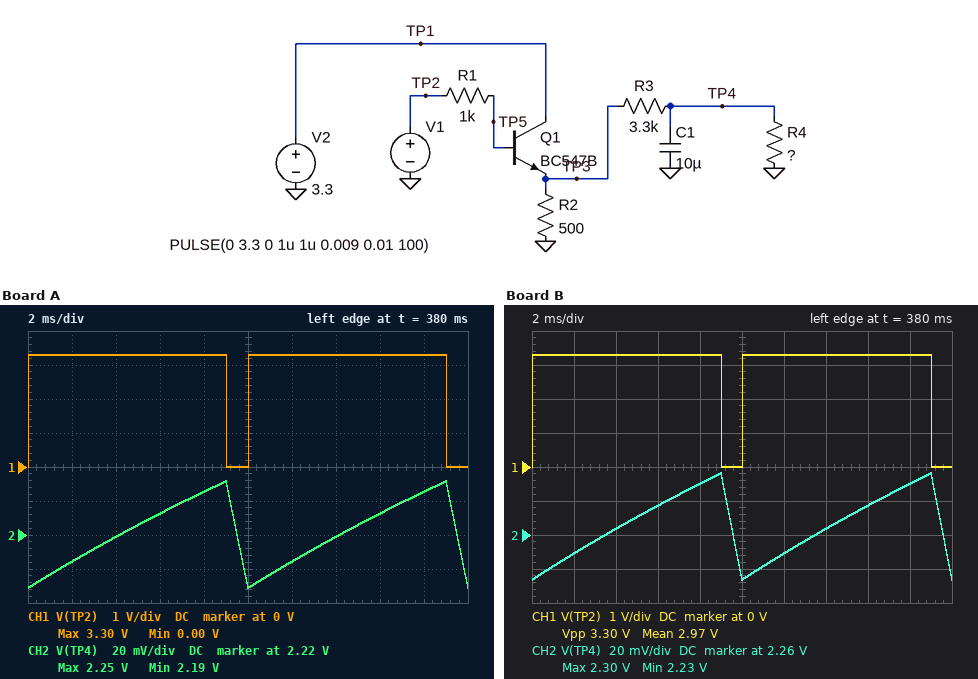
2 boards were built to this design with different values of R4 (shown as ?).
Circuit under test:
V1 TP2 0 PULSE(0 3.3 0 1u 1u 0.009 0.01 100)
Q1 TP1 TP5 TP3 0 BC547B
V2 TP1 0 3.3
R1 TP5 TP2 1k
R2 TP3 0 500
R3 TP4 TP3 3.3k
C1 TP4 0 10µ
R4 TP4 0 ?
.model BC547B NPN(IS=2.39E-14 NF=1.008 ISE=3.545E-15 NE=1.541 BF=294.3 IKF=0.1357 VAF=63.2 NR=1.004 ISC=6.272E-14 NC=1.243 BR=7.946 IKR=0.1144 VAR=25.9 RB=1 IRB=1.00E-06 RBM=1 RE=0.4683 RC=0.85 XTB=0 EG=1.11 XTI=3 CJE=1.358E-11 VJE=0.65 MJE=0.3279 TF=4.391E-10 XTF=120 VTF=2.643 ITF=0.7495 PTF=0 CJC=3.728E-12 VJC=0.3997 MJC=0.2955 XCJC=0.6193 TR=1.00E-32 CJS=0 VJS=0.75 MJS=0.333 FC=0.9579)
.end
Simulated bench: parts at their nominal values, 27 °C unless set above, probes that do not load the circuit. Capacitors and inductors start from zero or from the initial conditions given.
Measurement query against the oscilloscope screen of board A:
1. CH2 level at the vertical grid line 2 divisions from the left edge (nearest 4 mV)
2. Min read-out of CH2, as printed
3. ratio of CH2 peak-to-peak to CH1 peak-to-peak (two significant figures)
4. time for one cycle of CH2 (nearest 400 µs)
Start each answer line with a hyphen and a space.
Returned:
- 2.220 V
- 2.19 V
- 0.019
- 10.0 ms
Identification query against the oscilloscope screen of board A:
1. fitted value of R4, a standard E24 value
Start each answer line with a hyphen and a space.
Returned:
- 51 kΩ
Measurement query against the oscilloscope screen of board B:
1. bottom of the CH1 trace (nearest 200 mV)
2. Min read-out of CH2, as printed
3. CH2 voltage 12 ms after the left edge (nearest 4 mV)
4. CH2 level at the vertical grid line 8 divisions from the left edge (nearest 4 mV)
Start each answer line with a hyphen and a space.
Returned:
- 0 V
- 2.23 V
- 2.248 V
- 2.276 V
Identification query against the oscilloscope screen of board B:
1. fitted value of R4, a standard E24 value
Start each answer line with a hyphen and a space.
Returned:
- 75 kΩ
